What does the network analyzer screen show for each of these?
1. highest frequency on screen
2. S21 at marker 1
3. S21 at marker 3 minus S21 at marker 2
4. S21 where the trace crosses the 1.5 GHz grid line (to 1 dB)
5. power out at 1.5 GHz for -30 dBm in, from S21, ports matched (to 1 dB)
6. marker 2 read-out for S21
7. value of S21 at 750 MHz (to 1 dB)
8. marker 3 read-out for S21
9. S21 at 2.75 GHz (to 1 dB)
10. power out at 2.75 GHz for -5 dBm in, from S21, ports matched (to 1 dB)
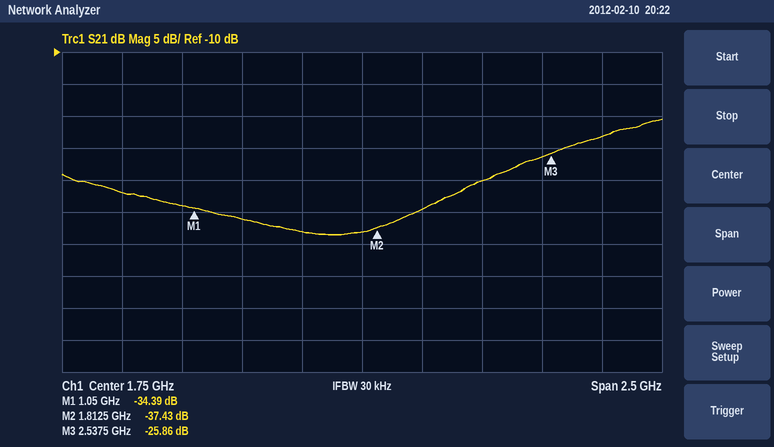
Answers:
3 GHz
-34.39 dB
11.57 dB
-38 dB
-68 dBm
-37.43 dB
-32 dB
-25.86 dB
-23 dB
-28 dBm
